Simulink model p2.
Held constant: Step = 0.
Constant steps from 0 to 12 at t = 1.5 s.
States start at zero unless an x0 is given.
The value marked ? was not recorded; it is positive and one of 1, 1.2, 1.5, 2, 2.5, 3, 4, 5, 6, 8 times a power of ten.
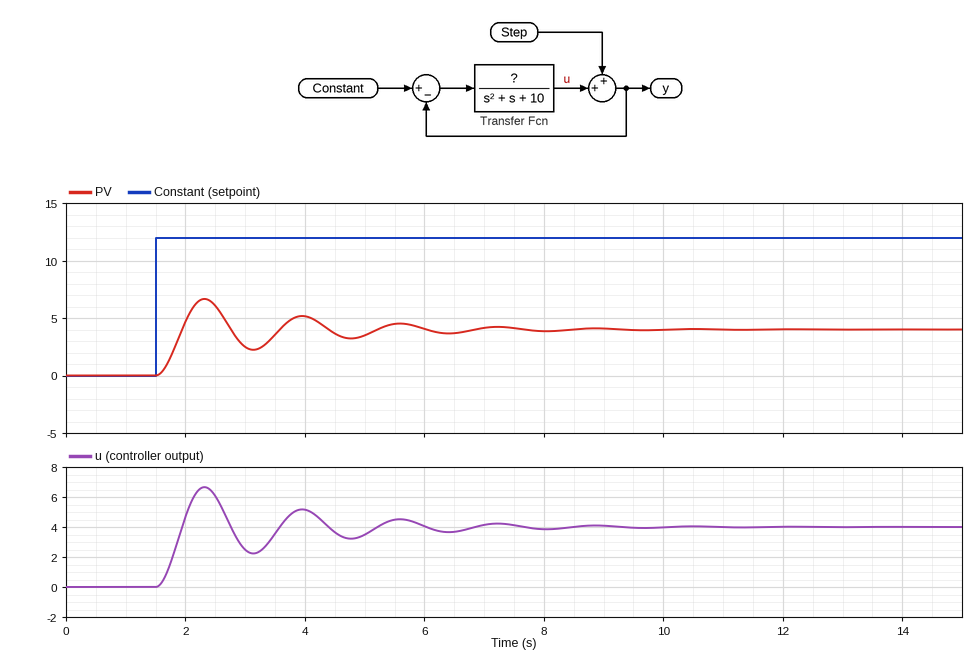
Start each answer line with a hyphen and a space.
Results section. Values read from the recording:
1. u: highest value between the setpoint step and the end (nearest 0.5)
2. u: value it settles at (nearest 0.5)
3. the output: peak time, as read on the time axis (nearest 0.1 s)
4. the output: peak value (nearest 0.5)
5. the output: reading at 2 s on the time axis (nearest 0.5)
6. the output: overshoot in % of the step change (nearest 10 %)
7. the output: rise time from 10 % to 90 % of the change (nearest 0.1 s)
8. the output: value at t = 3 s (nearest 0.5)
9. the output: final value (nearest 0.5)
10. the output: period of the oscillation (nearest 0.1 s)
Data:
- 6.5
- 4.0
- 2.3 s
- 6.5
- 4.5
- 70 %
- 0.3 s
- 2.5
- 4.0
- 1.6 s
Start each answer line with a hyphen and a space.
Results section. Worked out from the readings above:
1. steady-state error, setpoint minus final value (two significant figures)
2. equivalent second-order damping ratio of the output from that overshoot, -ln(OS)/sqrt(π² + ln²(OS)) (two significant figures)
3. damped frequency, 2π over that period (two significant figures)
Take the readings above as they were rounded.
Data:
- 8.0
- 0.11
- 3.9 rad/s
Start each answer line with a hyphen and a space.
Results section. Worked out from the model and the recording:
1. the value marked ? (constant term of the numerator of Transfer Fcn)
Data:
- 5
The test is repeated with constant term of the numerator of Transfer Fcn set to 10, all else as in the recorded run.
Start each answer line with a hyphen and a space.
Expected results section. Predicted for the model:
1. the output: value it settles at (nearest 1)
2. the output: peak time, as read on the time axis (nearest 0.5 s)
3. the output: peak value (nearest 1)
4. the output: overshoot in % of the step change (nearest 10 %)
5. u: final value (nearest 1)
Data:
- 6
- 2.0 s
- 10
- 70 %
- 6
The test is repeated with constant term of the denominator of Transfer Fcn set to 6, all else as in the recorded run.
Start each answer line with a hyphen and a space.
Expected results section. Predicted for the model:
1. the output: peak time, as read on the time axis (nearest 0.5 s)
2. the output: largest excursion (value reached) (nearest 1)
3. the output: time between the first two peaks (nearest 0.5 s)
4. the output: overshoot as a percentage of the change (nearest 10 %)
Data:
- 2.5 s
- 9
- 2.0 s
- 60 %
